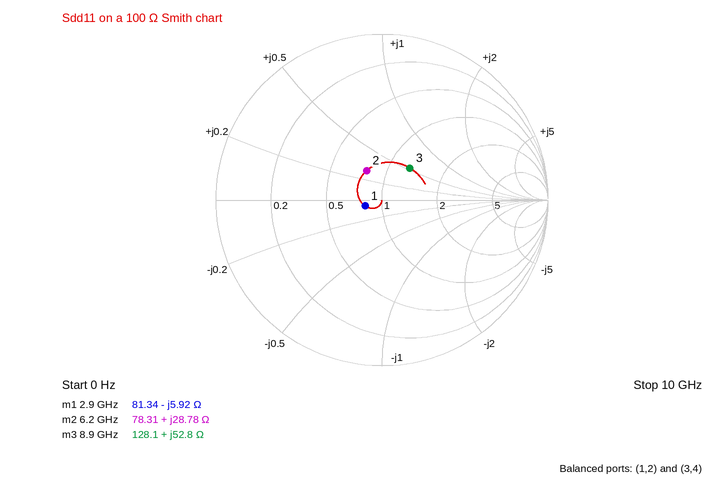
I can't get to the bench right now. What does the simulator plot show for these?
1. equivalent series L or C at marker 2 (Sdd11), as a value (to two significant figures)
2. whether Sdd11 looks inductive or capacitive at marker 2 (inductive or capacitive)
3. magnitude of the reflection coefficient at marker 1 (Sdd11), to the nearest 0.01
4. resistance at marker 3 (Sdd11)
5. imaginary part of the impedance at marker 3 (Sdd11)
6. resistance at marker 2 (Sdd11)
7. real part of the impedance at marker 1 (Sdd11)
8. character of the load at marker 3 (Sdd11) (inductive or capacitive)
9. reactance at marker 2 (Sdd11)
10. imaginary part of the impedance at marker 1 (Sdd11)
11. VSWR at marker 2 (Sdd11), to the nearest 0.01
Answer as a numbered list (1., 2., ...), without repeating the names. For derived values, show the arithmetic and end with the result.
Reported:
1. L = 28.78 Ω/(2π × 6.2 GHz) ≈ 739 pH, so 740 pH to two significant figures
2. inductive
3. 0.11
4. 128.1 Ω
5. +52.8 Ω
6. 78.31 Ω
7. 81.34 Ω
8. inductive
9. +28.78 Ω
10. -5.92 Ω
11. 1.50
